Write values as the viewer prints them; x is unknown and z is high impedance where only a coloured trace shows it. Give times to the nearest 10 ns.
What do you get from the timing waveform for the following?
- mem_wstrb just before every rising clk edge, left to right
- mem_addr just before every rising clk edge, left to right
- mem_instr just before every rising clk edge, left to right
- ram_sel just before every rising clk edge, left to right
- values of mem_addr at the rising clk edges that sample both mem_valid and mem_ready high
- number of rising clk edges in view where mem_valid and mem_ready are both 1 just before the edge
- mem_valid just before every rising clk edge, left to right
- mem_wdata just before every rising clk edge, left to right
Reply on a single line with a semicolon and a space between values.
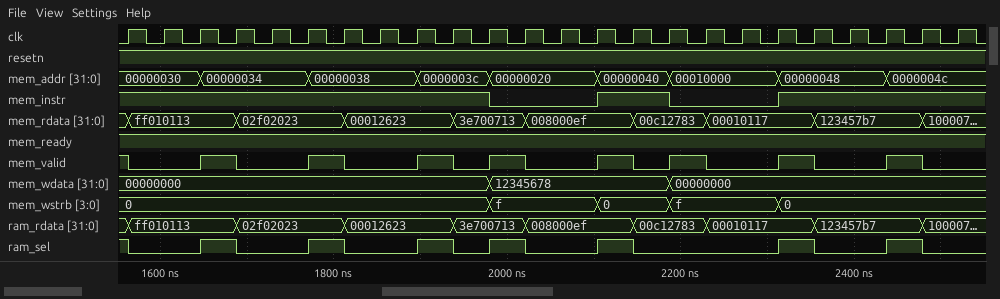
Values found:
0, 0, 0, 0, 0, 0, 0, 0, 0, 0, 0, f, f, f, 0, 0, f, f, f, 0, 0, 0, 0, 0; 00000030, 00000030, 00000030, 00000034, 00000034, 00000034, 00000038, 00000038, 00000038, 0000003c, 0000003c, 00000020, 00000020, 00000020, 00000040, 00000040, 00010000, 00010000, 00010000, 00000048, 00000048, 00000048, 0000004c, 0000004c; 1 1 1 1 1 1 1 1 1 1 1 0 0 0 1 1 0 0 0 1 1 1 1 1; 1 0 0 1 0 0 1 0 0 1 0 1 0 0 1 0 0 0 0 1 0 0 1 0; 00000030, 00000034, 00000038, 0000003c, 00000020, 00000040, 00010000, 00000048, 0000004c; 9; 1 0 0 1 0 0 1 0 0 1 0 1 0 0 1 0 1 0 0 1 0 0 1 0; 00000000, 00000000, 00000000, 00000000, 00000000, 00000000, 00000000, 00000000, 00000000, 00000000, 00000000, 12345678, 12345678, 12345678, 12345678, 12345678, 00000000, 00000000, 00000000, 00000000, 00000000, 00000000, 00000000, 00000000
